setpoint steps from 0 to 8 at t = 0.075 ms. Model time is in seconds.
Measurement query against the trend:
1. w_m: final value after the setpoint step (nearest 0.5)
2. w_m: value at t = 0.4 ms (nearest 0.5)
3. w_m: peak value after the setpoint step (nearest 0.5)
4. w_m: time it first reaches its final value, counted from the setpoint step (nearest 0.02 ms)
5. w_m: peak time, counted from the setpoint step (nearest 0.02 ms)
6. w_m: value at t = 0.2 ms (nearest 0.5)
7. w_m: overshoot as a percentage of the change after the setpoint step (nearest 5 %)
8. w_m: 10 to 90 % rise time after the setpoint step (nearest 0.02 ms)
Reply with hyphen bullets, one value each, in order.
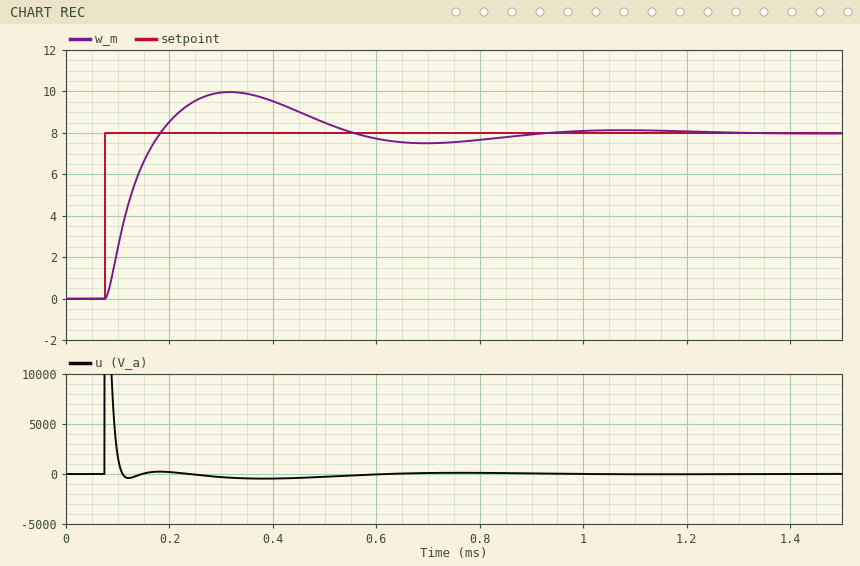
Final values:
- 8.0
- 9.5
- 10.0
- 0.10 ms
- 0.24 ms
- 8.5
- 25 %
- 0.08 ms
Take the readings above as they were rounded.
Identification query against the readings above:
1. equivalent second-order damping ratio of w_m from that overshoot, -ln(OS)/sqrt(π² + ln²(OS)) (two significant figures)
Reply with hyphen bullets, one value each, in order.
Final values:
- 0.40
